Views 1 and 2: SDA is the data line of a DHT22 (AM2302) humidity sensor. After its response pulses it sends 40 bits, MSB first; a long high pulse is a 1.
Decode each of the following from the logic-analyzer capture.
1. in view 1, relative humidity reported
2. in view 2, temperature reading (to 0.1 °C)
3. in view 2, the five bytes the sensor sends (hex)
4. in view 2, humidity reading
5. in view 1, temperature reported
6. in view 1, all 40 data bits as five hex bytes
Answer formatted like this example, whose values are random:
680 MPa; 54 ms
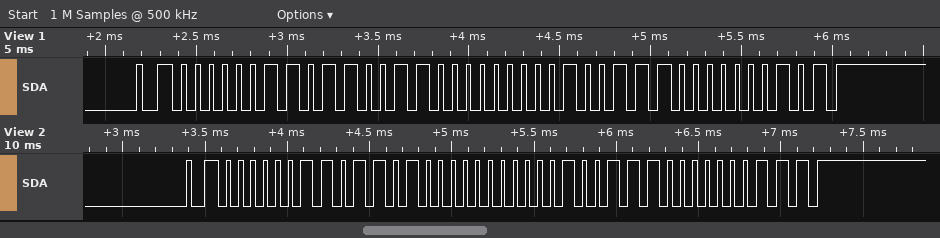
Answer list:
87.0 %; 15.6 °C; 03 68 00 9C 07; 87.2 %; 15.6 °C; 03 66 00 9C 05
